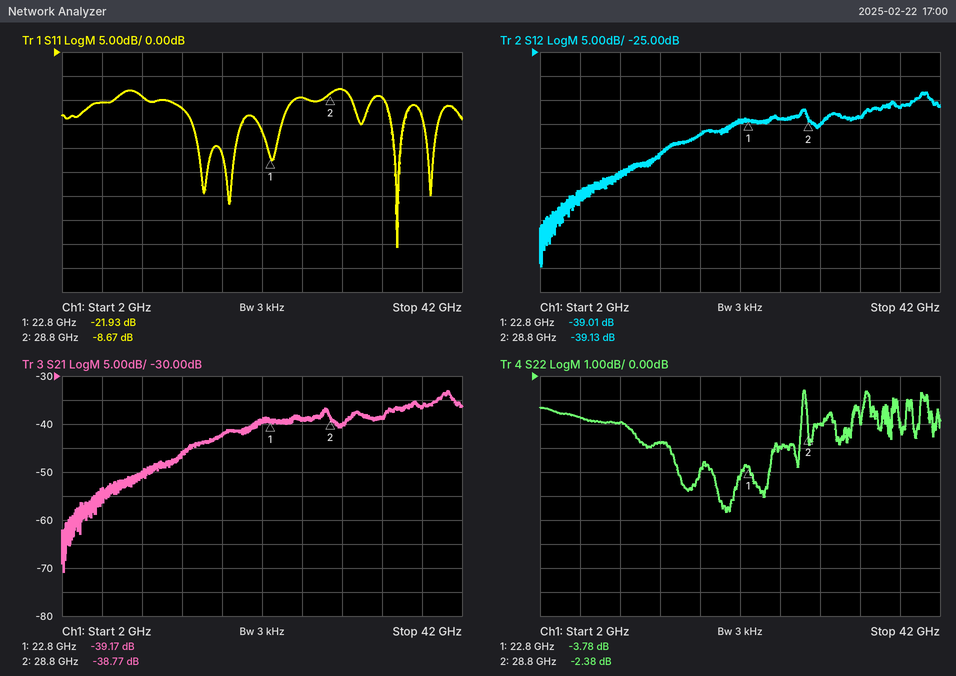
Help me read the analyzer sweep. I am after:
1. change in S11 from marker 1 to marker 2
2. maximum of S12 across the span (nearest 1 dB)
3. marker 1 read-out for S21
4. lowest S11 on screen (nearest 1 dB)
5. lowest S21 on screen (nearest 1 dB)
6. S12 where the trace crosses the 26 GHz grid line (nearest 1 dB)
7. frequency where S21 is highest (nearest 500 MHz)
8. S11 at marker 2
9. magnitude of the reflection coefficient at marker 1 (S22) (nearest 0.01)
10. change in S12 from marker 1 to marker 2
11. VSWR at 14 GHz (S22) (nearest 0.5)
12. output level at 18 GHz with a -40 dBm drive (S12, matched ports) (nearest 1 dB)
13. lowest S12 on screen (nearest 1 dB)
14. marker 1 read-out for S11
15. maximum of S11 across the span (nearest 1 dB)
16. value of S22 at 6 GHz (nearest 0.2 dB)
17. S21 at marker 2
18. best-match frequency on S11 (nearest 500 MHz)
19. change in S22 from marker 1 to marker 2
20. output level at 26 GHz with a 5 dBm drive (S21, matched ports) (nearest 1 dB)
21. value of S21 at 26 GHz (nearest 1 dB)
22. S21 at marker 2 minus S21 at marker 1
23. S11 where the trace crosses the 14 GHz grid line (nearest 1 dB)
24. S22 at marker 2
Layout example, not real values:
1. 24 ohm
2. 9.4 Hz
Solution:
1. 13.26 dB
2. -33 dB
3. -39.17 dB
4. -41 dB
5. -71 dB
6. -39 dB
7. 40.5 GHz
8. -8.67 dB
9. 0.65
10. -0.12 dB
11. 6.5
12. -82 dBm
13. -70 dB
14. -21.93 dB
15. -8 dB
16. -1.8 dB
17. -38.77 dB
18. 35.5 GHz
19. 1.40 dB
20. -34 dBm
21. -39 dB
22. 0.40 dB
23. -12 dB
24. -2.38 dB
